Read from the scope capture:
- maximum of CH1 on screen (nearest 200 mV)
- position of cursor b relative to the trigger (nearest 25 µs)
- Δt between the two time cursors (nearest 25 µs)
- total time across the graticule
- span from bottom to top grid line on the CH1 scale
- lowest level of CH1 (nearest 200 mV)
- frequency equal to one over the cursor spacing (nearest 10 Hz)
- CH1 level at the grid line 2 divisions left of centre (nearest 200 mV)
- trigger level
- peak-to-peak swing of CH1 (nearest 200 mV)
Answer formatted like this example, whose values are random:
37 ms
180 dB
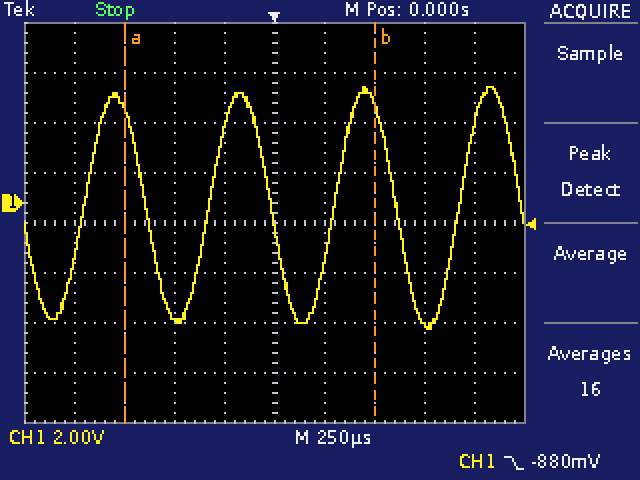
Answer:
4.6 V
+500 µs
1.250 ms
2.5 ms
16 V
-5.0 V
800 Hz
-4.6 V
-880 mV
9.6 V
